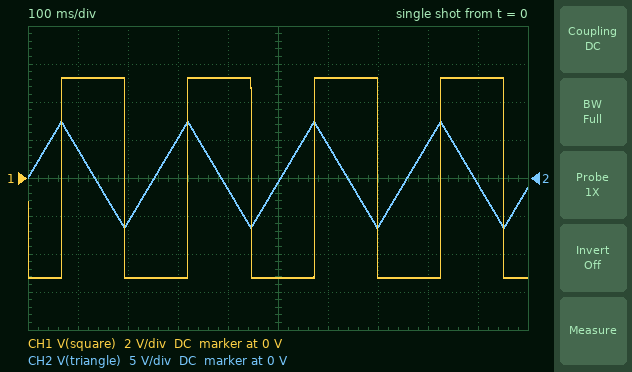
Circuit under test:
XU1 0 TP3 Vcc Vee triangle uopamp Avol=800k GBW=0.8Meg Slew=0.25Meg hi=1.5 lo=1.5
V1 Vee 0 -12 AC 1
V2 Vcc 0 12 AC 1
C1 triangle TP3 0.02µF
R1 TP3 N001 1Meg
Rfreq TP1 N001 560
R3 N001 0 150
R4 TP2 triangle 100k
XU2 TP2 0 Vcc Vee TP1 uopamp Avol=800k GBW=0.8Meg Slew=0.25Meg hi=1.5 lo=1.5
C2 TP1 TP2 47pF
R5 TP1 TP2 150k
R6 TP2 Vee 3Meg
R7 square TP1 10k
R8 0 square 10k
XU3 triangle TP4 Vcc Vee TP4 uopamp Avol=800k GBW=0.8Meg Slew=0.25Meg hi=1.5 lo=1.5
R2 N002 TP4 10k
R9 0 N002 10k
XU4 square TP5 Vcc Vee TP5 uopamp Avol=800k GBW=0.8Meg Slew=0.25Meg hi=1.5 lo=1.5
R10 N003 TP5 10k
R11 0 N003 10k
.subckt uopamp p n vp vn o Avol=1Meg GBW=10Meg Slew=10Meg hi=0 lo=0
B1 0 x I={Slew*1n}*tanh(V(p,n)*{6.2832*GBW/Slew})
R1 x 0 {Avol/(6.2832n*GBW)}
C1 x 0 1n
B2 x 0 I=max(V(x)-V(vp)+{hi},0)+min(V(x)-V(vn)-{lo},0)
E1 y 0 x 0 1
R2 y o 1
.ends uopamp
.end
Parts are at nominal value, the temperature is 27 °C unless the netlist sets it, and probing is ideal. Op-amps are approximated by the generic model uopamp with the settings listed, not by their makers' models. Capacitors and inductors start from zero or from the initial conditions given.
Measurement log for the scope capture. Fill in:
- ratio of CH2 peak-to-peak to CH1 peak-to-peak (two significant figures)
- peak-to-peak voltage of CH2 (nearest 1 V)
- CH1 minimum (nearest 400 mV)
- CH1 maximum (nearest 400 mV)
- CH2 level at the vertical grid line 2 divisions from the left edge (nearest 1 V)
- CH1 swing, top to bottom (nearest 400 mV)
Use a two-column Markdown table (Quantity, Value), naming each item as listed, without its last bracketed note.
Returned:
| Quantity | Value |
|---|---|
| ratio of CH2 peak-to-peak to CH1 peak-to-peak | 1.3 |
| peak-to-peak voltage of CH2 | 14 V |
| CH1 minimum | -5.2 V |
| CH1 maximum | 5.2 V |
| CH2 level at the vertical grid line 2 divisions from the left edge | -6 V |
| CH1 swing, top to bottom | 10.4 V |
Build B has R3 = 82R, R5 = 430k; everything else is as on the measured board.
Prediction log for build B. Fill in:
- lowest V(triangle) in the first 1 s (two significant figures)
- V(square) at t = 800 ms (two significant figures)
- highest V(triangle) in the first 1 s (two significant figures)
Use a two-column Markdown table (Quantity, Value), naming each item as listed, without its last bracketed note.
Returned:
| Quantity | Value |
|---|---|
| lowest V(triangle) in the first 1 s | -2.0 V |
| V(square) at t = 800 ms | 5.2 V |
| highest V(triangle) in the first 1 s | 2.8 V |
